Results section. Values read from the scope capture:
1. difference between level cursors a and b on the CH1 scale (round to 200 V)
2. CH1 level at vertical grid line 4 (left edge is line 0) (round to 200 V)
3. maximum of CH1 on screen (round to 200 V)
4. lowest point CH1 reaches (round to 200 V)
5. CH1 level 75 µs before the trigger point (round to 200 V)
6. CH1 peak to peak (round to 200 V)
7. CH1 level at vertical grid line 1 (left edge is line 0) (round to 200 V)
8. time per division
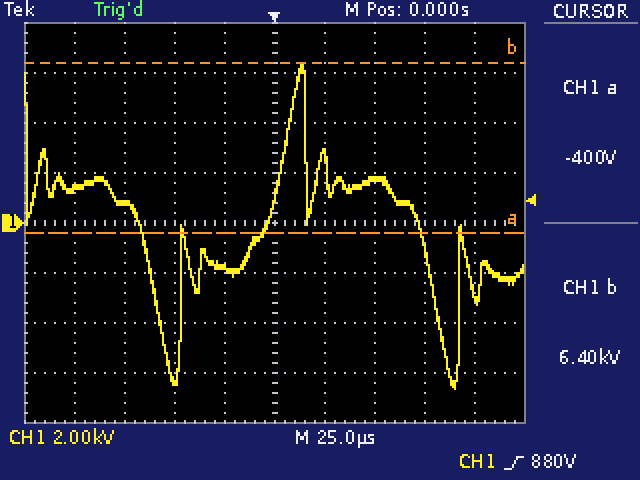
6.8 kV
-1.8 kV
6.4 kV
-6.6 kV
800 V
13.0 kV
1.4 kV
25 µs
